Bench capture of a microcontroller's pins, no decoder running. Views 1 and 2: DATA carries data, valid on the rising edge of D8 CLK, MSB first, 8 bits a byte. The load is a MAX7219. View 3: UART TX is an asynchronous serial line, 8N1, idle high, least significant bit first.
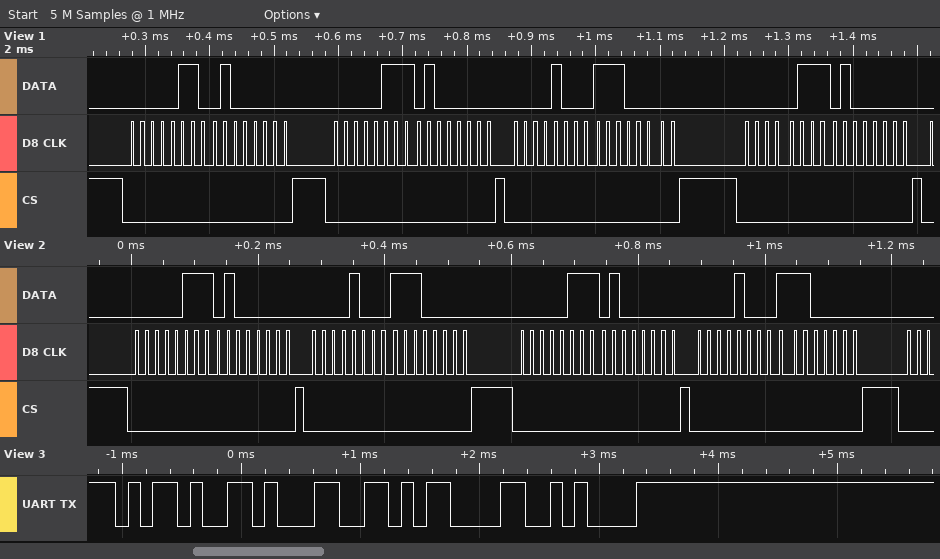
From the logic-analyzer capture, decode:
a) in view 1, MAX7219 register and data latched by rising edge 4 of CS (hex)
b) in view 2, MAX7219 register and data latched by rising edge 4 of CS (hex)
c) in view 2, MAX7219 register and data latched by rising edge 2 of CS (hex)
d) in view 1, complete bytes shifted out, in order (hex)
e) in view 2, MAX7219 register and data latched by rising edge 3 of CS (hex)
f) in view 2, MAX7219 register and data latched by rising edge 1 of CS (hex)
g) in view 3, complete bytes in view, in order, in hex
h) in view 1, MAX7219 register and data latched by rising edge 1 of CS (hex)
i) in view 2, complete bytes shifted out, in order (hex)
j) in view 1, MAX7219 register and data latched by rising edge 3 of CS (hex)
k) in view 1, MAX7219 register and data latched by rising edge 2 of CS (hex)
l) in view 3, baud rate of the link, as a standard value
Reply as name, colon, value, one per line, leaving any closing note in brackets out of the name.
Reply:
in view 1, MAX7219 register and data latched by rising edge 4 of CS: register 0x7, data 0x40
in view 2, MAX7219 register and data latched by rising edge 4 of CS: register 0x8, data 0xE0
in view 2, MAX7219 register and data latched by rising edge 2 of CS: register 0x8, data 0xE0
in view 1, complete bytes shifted out, in order: 06 40 07 40 08 E0 07 40
in view 2, MAX7219 register and data latched by rising edge 3 of CS: register 0x7, data 0x40
in view 2, MAX7219 register and data latched by rising edge 1 of CS: register 0x7, data 0x40
in view 3, complete bytes in view, in order, in hex: 2D 31 0D 0A
in view 1, MAX7219 register and data latched by rising edge 1 of CS: register 0x6, data 0x40
in view 2, complete bytes shifted out, in order: 07 40 08 E0 07 40 08 E0
in view 1, MAX7219 register and data latched by rising edge 3 of CS: register 0x8, data 0xE0
in view 1, MAX7219 register and data latched by rising edge 2 of CS: register 0x7, data 0x40
in view 3, baud rate of the link, as a standard value: 9600 baud
